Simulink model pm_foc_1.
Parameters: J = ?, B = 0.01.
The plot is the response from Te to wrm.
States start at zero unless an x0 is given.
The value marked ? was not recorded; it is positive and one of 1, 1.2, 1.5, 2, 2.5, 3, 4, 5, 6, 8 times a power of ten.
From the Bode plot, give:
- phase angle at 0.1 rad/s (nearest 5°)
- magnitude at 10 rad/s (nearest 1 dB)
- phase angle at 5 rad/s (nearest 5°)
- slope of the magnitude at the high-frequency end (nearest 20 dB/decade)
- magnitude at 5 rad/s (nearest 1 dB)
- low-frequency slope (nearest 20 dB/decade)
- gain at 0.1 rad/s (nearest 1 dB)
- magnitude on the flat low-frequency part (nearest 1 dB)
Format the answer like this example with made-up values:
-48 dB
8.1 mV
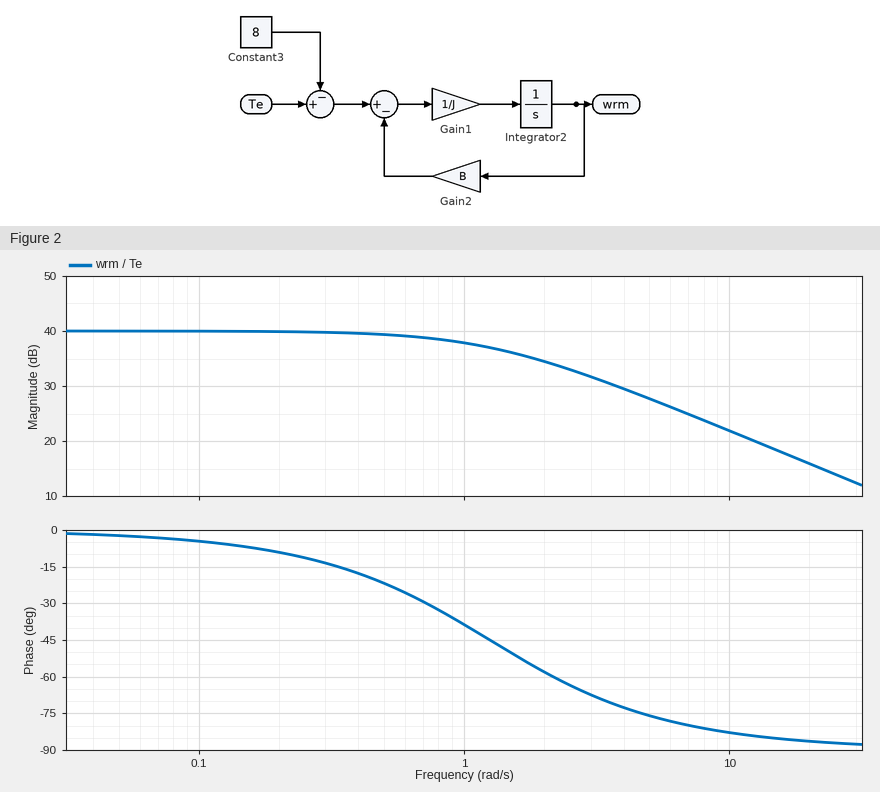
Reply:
-5°
22 dB
-75°
-20 dB/decade
28 dB
0 dB/decade
40 dB
40 dB
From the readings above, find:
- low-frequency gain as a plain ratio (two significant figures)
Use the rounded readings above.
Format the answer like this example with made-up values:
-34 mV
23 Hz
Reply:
100
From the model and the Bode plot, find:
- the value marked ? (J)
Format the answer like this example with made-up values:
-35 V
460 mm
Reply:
0.008
